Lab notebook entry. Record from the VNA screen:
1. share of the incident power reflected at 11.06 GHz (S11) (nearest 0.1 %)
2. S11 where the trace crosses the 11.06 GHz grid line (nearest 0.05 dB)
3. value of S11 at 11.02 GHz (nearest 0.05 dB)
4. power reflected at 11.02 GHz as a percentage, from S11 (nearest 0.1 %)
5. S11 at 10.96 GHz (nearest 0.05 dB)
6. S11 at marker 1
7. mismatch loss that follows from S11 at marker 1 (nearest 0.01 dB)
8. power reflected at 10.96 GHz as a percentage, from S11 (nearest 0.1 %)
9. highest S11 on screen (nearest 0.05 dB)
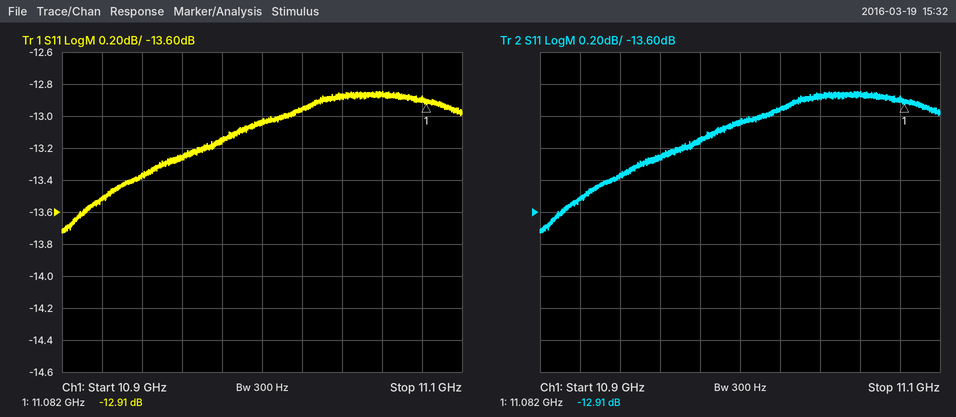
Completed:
5.2 %
-12.85 dB
-12.95 dB
5.1 %
-13.25 dB
-12.91 dB
0.23 dB
4.7 %
-12.85 dB
